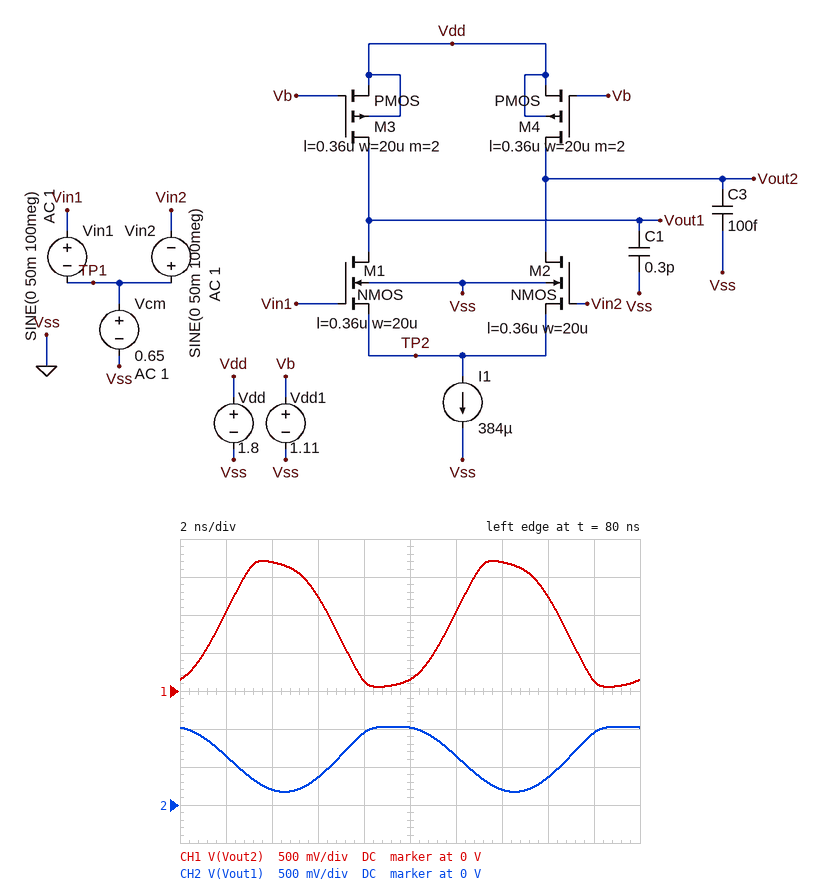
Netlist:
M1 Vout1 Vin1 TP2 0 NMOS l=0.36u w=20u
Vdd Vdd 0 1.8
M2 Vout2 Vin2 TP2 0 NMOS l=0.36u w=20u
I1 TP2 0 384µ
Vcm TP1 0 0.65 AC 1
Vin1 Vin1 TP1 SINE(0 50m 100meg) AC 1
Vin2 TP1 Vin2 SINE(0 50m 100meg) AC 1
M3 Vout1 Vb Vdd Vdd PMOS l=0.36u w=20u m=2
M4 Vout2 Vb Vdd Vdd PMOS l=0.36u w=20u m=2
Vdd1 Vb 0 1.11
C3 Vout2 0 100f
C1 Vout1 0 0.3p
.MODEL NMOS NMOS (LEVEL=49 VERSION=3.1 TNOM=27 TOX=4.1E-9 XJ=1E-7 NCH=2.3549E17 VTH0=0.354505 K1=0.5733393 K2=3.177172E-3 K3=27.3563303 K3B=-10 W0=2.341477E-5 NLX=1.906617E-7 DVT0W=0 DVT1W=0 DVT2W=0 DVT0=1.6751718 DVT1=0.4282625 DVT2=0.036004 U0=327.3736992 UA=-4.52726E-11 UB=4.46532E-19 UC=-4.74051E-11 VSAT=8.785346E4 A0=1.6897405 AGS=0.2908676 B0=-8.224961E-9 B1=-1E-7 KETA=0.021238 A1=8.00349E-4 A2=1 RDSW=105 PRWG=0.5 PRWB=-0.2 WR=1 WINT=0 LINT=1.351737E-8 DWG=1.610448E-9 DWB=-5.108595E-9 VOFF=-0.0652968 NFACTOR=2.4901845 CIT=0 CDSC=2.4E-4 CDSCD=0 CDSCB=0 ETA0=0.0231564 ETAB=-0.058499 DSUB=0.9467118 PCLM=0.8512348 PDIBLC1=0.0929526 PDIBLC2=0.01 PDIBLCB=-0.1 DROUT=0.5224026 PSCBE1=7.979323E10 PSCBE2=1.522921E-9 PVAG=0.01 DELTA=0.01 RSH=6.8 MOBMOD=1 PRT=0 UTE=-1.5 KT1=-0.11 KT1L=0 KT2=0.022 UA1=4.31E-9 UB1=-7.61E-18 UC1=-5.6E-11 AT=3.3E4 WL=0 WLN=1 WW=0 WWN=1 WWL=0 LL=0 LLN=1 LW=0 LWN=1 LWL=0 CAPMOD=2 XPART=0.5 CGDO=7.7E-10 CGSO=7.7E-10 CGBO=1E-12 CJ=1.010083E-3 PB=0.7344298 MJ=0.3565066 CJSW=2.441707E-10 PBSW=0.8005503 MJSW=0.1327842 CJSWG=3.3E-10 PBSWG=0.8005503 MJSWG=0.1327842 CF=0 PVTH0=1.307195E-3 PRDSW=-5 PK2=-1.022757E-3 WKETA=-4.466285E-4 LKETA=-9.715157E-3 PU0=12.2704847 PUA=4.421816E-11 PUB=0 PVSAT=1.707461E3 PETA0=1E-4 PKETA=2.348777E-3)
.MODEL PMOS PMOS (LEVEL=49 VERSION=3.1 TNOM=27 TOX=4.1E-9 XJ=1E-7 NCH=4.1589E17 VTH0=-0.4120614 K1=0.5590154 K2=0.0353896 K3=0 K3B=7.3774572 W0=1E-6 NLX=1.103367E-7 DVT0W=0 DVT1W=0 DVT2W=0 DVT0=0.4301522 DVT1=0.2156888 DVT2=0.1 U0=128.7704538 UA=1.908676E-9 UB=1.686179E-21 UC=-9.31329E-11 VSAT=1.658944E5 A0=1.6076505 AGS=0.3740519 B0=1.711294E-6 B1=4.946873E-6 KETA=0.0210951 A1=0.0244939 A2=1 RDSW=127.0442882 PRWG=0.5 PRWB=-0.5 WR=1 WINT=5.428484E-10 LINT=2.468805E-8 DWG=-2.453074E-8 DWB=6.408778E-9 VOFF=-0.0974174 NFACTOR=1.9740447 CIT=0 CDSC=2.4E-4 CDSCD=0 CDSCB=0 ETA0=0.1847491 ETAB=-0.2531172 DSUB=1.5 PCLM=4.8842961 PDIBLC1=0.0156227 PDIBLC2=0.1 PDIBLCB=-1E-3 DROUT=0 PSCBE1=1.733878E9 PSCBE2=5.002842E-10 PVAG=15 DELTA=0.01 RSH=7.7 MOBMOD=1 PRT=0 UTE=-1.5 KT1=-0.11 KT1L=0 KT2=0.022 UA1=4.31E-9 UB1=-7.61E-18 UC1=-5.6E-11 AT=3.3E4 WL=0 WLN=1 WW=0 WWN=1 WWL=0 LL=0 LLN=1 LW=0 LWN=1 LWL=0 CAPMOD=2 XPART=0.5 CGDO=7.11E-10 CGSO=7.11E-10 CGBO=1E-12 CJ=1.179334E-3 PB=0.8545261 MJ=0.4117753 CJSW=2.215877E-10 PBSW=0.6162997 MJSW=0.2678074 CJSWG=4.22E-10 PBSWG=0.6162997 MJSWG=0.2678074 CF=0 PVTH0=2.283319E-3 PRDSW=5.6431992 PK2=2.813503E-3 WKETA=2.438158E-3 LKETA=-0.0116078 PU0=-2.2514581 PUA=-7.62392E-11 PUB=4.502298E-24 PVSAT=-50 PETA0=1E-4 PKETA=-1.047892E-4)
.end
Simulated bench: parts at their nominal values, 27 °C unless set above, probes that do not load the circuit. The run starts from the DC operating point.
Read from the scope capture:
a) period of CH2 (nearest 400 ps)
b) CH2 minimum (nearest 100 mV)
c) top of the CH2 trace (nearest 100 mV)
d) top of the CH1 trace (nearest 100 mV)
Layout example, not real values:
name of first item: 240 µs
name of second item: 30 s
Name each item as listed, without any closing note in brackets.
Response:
period of CH2: 10.0 ns
CH2 minimum: 200 mV
top of the CH2 trace: 1.0 V
top of the CH1 trace: 1.7 V
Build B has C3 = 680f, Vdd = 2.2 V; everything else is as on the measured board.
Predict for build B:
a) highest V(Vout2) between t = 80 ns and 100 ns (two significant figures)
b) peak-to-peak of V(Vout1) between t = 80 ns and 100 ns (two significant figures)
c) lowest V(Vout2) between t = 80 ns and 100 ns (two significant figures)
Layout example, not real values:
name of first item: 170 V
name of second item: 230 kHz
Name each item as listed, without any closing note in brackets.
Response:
highest V(Vout2) between t = 80 ns and 100 ns: 2.2 V
peak-to-peak of V(Vout1) between t = 80 ns and 100 ns: 52 mV
lowest V(Vout2) between t = 80 ns and 100 ns: 2.1 V
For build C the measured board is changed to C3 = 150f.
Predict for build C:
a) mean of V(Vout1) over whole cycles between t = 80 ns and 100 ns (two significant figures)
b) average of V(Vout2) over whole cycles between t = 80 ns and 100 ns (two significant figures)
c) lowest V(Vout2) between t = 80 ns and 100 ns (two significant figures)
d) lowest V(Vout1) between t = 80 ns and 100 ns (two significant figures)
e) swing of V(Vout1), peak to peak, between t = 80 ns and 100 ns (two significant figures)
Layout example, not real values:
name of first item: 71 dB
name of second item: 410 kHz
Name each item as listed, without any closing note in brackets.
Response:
mean of V(Vout1) over whole cycles between t = 80 ns and 100 ns: 860 mV
average of V(Vout2) over whole cycles between t = 80 ns and 100 ns: 890 mV
lowest V(Vout2) between t = 80 ns and 100 ns: 120 mV
lowest V(Vout1) between t = 80 ns and 100 ns: 360 mV
swing of V(Vout1), peak to peak, between t = 80 ns and 100 ns: 980 mV
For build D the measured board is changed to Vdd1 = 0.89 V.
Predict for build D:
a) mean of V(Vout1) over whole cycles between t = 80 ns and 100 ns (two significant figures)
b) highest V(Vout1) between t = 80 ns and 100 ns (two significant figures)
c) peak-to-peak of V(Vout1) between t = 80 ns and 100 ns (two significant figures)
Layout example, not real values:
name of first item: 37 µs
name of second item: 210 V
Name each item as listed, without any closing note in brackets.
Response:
mean of V(Vout1) over whole cycles between t = 80 ns and 100 ns: 1.7 V
highest V(Vout1) between t = 80 ns and 100 ns: 1.8 V
peak-to-peak of V(Vout1) between t = 80 ns and 100 ns: 76 mV
